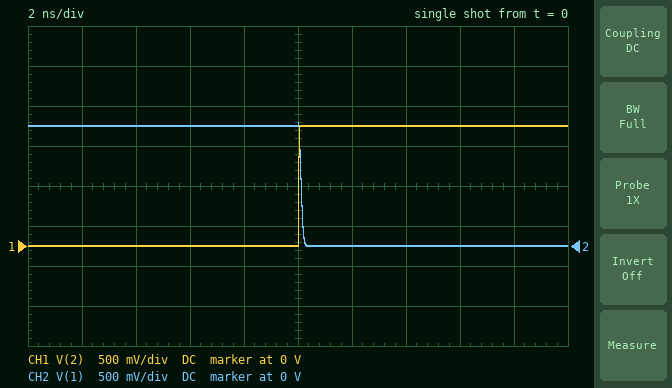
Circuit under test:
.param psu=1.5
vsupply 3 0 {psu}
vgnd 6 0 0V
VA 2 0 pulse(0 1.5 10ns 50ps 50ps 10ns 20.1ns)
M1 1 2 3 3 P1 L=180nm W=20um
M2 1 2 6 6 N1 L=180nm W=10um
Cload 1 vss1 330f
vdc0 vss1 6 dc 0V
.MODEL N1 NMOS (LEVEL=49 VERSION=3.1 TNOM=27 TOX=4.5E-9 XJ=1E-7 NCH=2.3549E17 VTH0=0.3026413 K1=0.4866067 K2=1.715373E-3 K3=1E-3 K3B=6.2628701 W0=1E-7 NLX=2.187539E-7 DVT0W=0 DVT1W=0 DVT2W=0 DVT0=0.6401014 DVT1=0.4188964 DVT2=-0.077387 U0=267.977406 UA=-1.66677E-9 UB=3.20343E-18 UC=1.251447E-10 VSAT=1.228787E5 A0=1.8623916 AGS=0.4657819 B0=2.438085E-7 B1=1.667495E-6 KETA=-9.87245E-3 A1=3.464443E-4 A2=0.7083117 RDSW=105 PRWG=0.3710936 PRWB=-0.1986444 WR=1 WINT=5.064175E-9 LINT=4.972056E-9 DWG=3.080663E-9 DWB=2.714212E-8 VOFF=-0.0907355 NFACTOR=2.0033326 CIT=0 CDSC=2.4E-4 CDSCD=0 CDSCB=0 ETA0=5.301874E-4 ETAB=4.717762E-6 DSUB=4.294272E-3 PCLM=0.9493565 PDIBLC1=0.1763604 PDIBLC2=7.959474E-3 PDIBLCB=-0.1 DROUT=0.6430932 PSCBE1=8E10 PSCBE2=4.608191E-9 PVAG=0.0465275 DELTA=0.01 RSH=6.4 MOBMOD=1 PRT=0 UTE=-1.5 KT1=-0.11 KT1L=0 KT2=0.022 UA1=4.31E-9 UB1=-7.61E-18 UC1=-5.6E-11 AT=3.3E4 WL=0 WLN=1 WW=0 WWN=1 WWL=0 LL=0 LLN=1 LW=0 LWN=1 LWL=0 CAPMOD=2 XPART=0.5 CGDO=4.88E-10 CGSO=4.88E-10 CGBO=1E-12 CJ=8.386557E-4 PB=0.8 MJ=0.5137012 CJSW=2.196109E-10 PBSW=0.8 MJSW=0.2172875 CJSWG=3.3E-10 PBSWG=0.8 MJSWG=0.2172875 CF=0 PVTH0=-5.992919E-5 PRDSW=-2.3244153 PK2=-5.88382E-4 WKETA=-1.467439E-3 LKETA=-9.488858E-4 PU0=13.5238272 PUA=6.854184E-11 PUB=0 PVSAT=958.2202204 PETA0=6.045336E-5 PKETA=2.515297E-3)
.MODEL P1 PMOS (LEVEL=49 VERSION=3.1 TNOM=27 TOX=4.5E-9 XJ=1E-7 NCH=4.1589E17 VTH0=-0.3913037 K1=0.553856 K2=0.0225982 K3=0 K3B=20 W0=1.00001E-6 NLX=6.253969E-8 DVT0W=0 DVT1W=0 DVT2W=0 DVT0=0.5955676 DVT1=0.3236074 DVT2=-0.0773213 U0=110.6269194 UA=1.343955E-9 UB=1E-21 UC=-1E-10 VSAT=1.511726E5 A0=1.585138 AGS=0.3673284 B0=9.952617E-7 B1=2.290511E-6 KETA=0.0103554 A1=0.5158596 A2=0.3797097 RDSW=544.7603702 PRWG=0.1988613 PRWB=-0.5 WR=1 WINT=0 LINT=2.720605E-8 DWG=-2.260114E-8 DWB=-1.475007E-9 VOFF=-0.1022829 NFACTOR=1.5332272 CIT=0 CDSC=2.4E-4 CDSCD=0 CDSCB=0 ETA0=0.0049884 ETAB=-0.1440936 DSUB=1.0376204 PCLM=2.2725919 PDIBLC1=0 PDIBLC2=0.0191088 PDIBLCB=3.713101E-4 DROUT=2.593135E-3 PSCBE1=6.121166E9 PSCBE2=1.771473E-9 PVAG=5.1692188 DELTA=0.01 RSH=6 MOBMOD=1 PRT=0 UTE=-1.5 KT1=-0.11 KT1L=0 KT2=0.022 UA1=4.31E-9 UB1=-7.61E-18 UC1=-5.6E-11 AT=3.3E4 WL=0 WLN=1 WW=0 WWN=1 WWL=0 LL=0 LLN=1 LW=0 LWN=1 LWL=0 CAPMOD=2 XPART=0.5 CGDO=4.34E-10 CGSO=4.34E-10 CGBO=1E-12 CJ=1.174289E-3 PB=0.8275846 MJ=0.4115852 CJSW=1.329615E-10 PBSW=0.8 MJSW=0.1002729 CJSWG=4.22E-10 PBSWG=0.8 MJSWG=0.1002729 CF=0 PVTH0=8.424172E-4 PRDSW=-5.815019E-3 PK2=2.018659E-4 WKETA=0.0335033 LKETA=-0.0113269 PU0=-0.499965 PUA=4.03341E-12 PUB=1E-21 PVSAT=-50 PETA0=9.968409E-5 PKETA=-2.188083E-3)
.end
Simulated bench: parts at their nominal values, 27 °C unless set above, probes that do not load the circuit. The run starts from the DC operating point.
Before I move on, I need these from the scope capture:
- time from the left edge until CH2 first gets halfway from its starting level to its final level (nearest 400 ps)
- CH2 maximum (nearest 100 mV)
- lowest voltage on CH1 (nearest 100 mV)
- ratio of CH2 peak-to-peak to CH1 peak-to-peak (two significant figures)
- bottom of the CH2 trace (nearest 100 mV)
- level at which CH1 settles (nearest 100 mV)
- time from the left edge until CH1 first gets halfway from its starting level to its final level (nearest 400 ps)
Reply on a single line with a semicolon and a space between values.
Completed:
10.0 ns; 1.5 V; 0 V; 1.0; 0 V; 1.5 V; 10.0 ns
